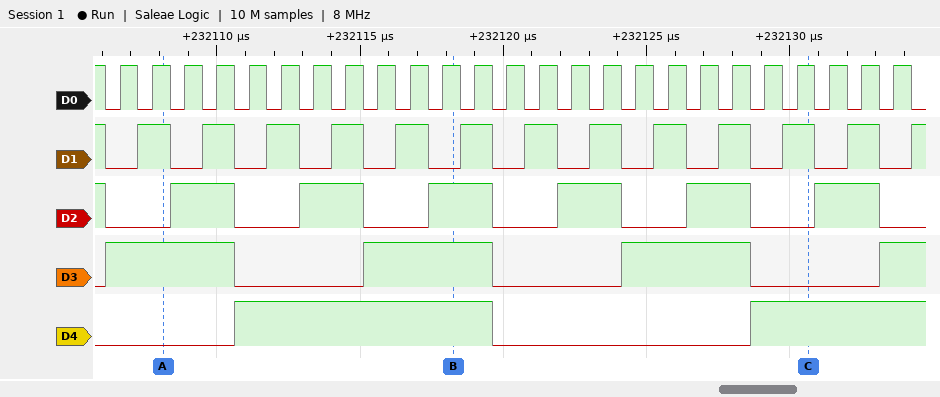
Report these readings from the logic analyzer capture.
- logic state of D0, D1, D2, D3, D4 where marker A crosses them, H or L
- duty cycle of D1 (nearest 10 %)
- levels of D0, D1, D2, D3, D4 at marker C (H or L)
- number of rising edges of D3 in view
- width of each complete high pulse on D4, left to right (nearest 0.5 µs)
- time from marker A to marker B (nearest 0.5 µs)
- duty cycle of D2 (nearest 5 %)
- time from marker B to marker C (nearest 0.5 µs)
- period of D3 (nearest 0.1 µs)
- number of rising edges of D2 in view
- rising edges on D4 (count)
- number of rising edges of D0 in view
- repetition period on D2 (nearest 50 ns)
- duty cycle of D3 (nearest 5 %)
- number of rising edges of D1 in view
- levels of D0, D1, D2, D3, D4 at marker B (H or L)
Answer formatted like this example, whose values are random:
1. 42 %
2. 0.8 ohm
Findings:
1. D0=H, D1=H, D2=L, D3=H, D4=L
2. 50 %
3. D0=H, D1=H, D2=L, D3=L, D4=H
4. 4
5. 9 µs
6. 10 µs
7. 50 %
8. 12.5 µs
9. 9 µs
10. 6
11. 2
12. 25
13. 4500 ns
14. 50 %
15. 13
16. D0=H, D1=L, D2=H, D3=H, D4=H
